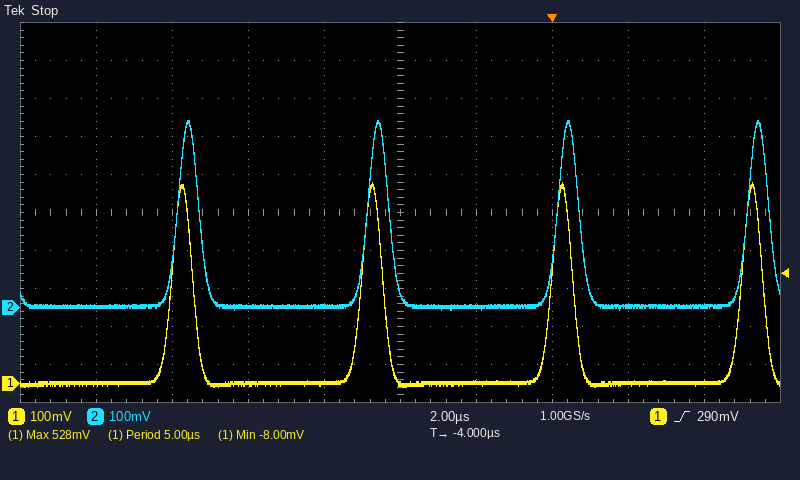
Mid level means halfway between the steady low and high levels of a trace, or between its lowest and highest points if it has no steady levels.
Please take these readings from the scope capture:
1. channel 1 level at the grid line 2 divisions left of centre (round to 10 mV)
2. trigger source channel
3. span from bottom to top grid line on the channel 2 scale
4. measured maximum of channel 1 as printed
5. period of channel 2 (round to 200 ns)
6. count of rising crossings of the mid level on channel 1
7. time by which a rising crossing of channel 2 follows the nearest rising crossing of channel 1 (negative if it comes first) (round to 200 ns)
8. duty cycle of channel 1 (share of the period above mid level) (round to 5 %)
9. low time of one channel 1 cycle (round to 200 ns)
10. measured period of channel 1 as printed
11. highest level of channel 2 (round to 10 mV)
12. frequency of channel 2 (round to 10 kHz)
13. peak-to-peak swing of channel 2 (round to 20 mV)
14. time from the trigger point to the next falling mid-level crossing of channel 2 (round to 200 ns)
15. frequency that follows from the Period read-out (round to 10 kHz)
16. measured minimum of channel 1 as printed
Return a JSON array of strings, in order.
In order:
["0 mV", "channel 1", "1 V", "528 mV", "5.0 µs", "4", "+200 ns", "10 %", "4.4 µs", "5.00 µs", "490 mV", "200 kHz", "500 mV", "800 ns", "200 kHz", "-8.00 mV"]
